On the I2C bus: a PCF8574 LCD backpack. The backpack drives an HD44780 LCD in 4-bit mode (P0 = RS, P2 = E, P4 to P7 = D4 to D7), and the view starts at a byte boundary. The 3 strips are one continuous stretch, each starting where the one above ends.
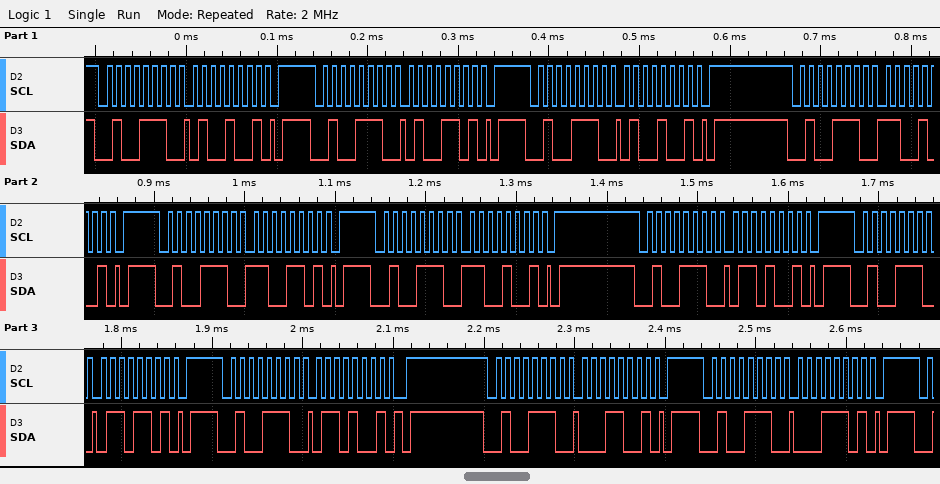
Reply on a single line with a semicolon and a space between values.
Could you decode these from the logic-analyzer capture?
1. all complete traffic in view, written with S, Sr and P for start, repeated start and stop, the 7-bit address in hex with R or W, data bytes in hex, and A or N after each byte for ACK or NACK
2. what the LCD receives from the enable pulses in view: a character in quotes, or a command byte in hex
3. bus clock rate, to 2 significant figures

S 27W A 49 A P S 27W A 4D A P S 27W A 49 A P S 27W A C9 A P S 27W A CD A P S 27W A C9 A P S 27W A 69 A P S 27W A 6D A P S 27W A 69 A P S 27W A 19 A P S 27W A 1D A P; 'L'; 100 kHz
